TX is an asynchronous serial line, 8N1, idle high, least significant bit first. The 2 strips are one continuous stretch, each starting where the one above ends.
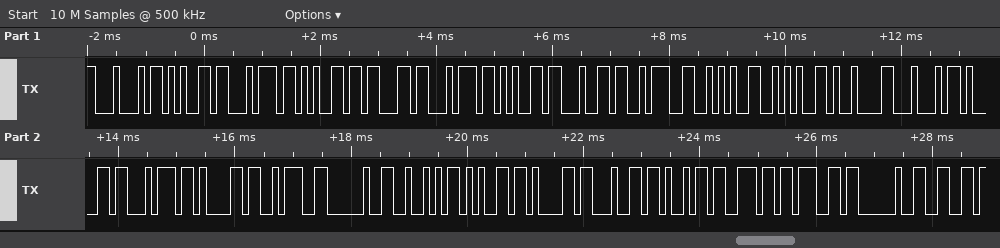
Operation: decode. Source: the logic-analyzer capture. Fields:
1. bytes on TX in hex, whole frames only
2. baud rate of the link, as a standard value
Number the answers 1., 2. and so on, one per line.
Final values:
1. 0x44 0x65 0x74 0x65 0x63 0x74 0x65 0x64 0x3A 0x2A 0x2A 0x09 0x44 0x61 0x74 0x61 0x3A 0x20 0x52 0x65 0x61 0x64 0x69 0x6E 0x67 0x20 0x66
2. 9600 baud
